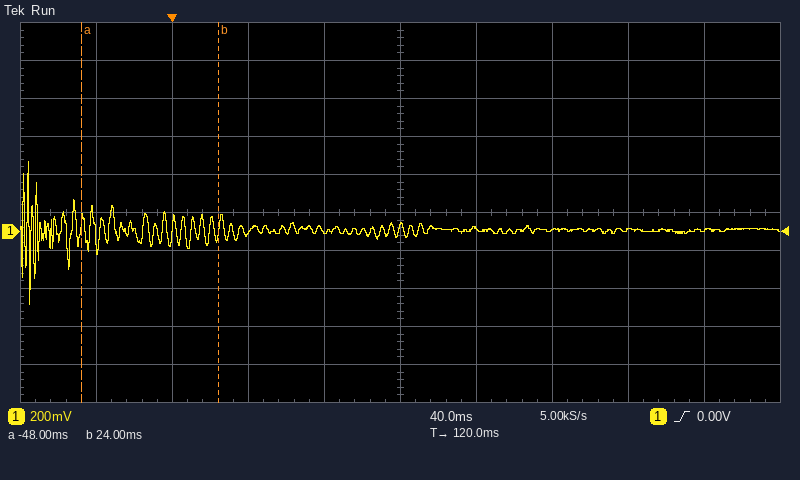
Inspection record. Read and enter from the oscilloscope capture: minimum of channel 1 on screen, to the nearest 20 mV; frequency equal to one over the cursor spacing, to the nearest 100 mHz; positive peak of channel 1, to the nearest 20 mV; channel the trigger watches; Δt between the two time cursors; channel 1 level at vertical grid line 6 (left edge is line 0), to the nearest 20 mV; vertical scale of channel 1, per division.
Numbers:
-380 mV
13.9 Hz
360 mV
channel 1
72 ms
20 mV
200 mV
